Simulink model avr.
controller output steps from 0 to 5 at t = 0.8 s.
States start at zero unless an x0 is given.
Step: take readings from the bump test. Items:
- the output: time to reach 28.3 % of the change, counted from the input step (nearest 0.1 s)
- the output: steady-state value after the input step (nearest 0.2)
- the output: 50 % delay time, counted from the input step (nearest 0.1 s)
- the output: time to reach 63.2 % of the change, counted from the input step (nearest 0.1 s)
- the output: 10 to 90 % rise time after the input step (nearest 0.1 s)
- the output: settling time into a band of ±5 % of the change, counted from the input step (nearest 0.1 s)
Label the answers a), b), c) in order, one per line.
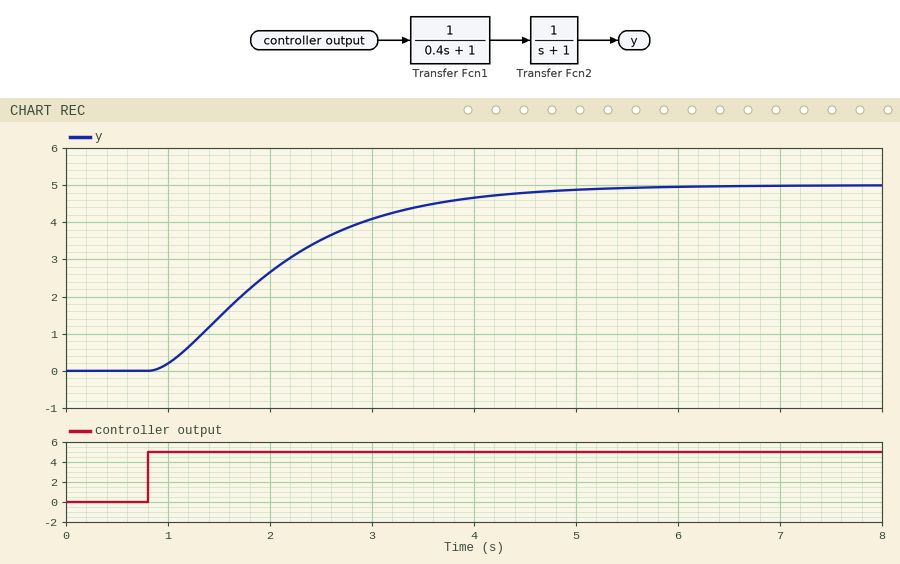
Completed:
a) 0.7 s
b) 5.0
c) 1.1 s
d) 1.5 s
e) 2.5 s
f) 3.5 s
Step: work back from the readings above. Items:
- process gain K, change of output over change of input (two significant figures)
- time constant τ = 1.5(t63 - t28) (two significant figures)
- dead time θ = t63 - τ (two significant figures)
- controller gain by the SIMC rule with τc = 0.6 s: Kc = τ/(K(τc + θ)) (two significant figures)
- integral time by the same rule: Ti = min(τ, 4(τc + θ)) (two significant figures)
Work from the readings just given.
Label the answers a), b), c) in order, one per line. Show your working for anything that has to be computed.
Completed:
a) (5 - 0) / 5 = 1.0
b) 1.5 × (1.5 - 0.7) = 1.2 s
c) 1.5 - 1.2 = 0.30 s
d) 1.2 / (1 × (0.6 + 0.3)) = 1.3
e) min(1.2, 4 × (0.6 + 0.3)) = 1.2 s
